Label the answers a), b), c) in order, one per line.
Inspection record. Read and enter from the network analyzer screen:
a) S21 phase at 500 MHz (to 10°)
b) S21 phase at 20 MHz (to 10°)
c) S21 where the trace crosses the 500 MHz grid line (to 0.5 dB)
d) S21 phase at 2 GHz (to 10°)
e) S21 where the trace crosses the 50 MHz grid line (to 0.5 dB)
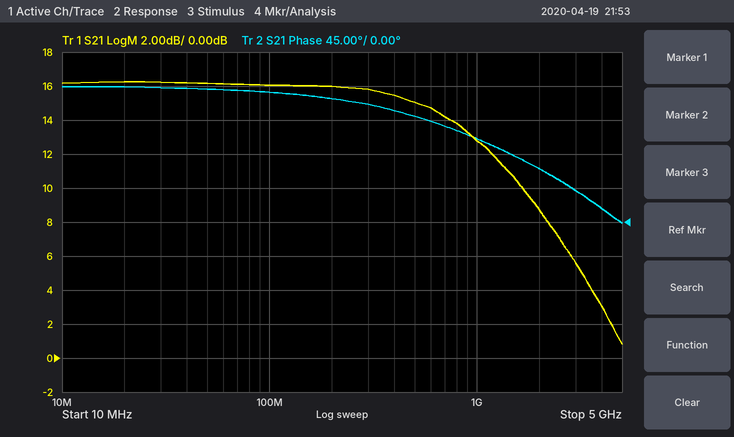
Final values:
a) 140°
b) 180°
c) 15.0 dB
d) 70°
e) 16.0 dB
